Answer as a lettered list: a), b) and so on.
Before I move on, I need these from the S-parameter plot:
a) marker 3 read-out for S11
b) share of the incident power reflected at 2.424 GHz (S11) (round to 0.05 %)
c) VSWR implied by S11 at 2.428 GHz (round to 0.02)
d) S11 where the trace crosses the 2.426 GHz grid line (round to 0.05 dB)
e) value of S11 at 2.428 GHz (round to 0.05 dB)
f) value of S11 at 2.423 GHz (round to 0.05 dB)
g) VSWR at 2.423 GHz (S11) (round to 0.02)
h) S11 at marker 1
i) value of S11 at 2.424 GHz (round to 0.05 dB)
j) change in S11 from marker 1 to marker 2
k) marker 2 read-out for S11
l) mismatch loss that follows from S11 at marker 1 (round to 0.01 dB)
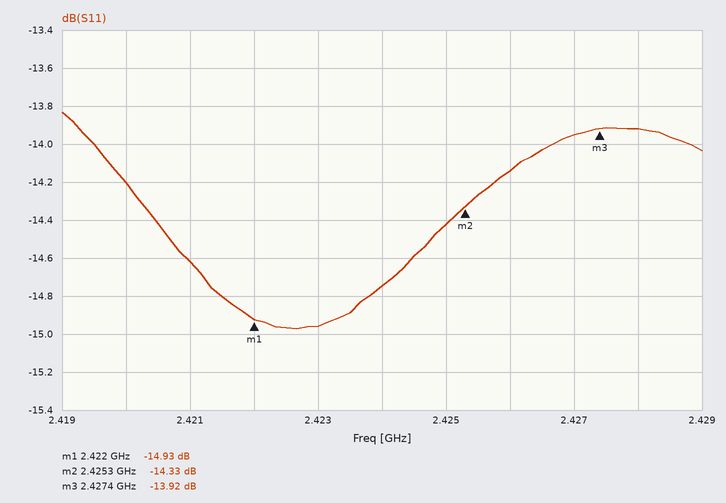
a) -13.92 dB
b) 3.35 %
c) 1.50
d) -14.15 dB
e) -13.90 dB
f) -14.95 dB
g) 1.44
h) -14.93 dB
i) -14.75 dB
j) 0.60 dB
k) -14.33 dB
l) 0.14 dB
